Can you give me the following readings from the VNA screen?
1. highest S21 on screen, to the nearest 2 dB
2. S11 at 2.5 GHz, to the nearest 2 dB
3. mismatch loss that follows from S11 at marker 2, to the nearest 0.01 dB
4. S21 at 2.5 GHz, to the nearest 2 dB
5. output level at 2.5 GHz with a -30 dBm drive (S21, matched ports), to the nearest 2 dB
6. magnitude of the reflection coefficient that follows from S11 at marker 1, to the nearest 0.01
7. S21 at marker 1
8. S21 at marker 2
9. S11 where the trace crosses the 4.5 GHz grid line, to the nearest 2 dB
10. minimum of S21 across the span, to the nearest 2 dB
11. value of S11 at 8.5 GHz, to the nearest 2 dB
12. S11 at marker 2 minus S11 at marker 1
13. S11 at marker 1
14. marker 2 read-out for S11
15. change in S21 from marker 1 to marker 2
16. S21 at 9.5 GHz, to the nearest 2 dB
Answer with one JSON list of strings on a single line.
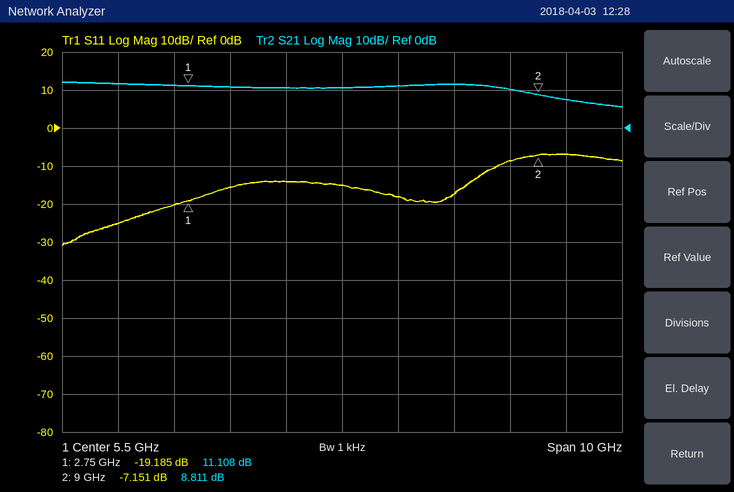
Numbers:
["12 dB", "-20 dB", "0.93 dB", "12 dB", "-18 dBm", "0.11", "11.108 dB", "8.811 dB", "-14 dB", "6 dB", "-8 dB", "12.034 dB", "-19.185 dB", "-7.151 dB", "-2.297 dB", "8 dB"]
